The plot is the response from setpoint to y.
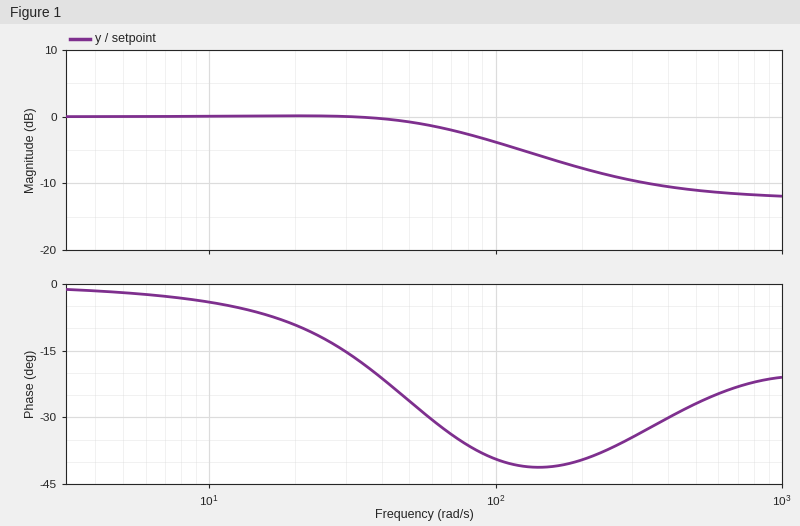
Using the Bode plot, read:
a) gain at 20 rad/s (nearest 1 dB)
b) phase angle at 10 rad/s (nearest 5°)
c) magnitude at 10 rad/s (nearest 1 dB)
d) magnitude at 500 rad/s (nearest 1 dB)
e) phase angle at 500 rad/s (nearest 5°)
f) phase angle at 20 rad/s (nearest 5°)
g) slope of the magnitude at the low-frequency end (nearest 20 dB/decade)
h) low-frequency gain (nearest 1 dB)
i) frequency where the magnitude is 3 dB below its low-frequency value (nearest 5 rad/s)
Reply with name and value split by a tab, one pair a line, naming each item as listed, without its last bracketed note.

gain at 20 rad/s	0 dB
phase angle at 10 rad/s	-5°
magnitude at 10 rad/s	0 dB
magnitude at 500 rad/s	-11 dB
phase angle at 500 rad/s	-25°
phase angle at 20 rad/s	-10°
slope of the magnitude at the low-frequency end	0 dB/decade
low-frequency gain	0 dB
frequency where the magnitude is 3 dB below its low-frequency value	85 rad/s
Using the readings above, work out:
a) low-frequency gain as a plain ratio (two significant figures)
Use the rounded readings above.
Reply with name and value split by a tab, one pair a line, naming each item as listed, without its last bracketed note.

low-frequency gain as a plain ratio	1.0
